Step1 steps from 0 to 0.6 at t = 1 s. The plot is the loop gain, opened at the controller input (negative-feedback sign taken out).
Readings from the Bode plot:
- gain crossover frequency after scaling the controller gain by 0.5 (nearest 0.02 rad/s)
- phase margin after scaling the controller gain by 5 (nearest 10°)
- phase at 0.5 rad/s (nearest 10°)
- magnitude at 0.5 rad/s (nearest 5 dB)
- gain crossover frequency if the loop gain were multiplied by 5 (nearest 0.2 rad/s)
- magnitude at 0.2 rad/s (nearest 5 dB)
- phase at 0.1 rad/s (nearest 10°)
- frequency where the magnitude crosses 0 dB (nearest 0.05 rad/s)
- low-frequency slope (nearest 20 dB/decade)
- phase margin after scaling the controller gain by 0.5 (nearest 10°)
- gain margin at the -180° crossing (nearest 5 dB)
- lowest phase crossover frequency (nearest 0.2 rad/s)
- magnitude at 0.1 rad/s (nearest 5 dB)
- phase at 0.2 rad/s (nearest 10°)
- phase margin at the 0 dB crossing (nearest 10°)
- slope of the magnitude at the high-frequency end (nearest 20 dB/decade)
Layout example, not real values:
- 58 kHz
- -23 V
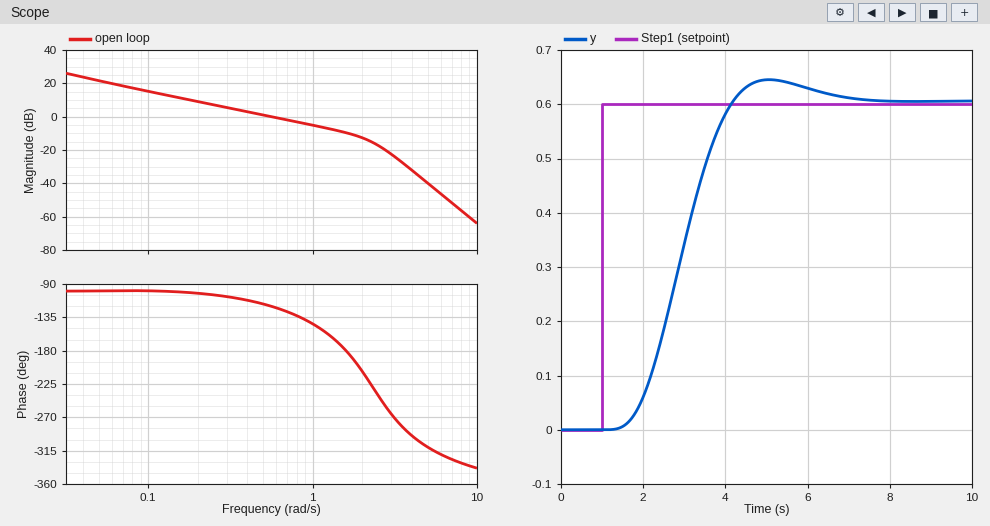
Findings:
- 0.28 rad/s
- -40°
- -120°
- 0 dB
- 2.2 rad/s
- 10 dB
- -100°
- 0.55 rad/s
- -20 dB/decade
- 70°
- 10 dB
- 1.6 rad/s
- 15 dB
- -100°
- 60°
- -80 dB/decade
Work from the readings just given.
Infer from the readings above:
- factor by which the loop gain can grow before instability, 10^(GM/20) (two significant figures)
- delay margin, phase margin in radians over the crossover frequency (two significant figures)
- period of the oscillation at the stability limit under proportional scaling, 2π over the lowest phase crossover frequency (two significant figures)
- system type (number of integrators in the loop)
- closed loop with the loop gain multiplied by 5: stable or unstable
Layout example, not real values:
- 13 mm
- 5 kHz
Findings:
- 3.2
- 1.9 s
- 3.9 s
- 1
- unstable
